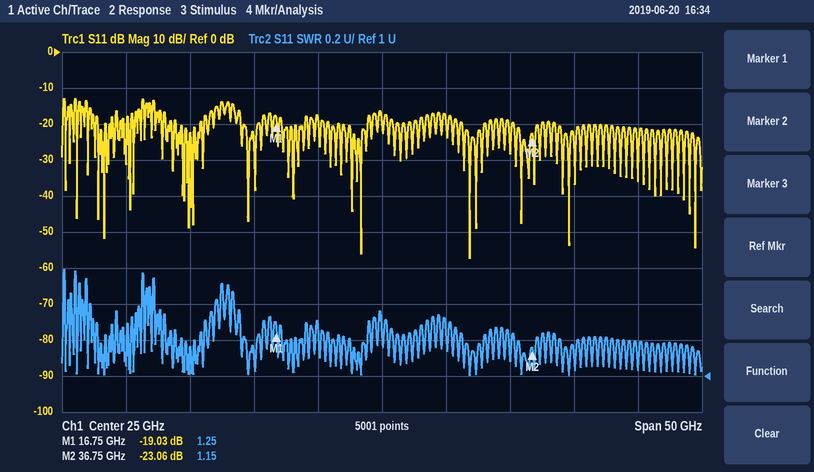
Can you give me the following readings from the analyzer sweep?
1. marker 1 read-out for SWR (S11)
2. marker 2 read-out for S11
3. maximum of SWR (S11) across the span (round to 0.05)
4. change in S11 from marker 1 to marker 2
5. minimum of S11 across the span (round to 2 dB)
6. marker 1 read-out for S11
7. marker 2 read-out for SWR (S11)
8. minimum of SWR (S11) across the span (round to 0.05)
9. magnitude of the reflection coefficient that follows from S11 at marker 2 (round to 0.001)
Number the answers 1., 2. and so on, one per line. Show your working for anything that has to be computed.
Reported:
1. 1.25
2. -23.06 dB
3. 1.60
4. -23.06 − (-19.03) = -4.03 dB
5. -58 dB
6. -19.03 dB
7. 1.15
8. 1.00
9. 10^(-23.06/20) ≈ 0.070
